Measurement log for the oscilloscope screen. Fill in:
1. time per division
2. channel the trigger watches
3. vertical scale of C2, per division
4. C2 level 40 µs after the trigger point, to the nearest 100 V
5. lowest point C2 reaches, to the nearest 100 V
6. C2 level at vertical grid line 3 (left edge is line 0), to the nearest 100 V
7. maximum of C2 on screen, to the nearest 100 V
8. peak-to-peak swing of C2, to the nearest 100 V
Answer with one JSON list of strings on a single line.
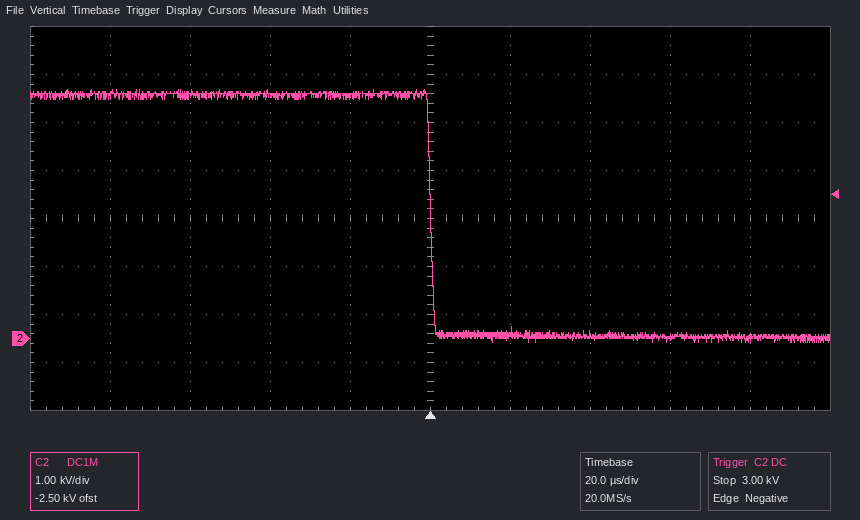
["20 µs", "C2", "1 kV", "100 V", "-100 V", "5.1 kV", "5.2 kV", "5.3 kV"]
